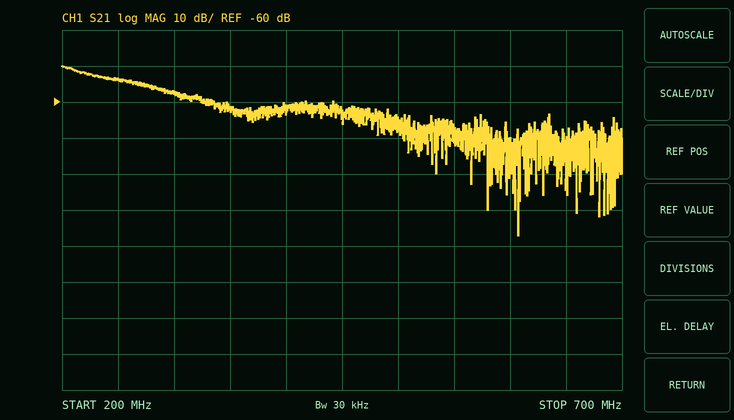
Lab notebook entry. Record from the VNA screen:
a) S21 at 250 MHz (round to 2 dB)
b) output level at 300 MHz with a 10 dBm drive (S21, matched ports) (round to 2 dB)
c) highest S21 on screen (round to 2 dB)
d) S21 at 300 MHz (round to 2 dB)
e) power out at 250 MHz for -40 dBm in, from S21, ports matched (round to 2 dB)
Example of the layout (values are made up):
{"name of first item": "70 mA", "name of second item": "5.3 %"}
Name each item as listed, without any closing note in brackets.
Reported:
{"S21 at 250 MHz": "-54 dB", "output level at 300 MHz with a 10 dBm drive (S21, matched ports)": "-48 dBm", "highest S21 on screen": "-50 dB", "S21 at 300 MHz": "-58 dB", "power out at 250 MHz for -40 dBm in, from S21, ports matched": "-94 dBm"}
